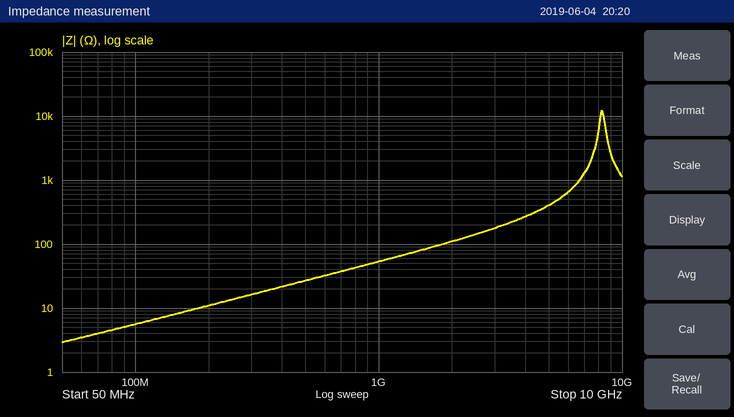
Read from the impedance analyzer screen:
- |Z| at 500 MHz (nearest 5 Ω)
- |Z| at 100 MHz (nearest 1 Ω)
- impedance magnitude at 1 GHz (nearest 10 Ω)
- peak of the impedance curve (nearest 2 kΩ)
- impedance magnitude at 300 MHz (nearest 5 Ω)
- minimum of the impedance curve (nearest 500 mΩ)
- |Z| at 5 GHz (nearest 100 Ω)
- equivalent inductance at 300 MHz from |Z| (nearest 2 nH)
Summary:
25 Ω
6 Ω
50 Ω
12 kΩ
15 Ω
3.0 Ω
400 Ω
8 nH
